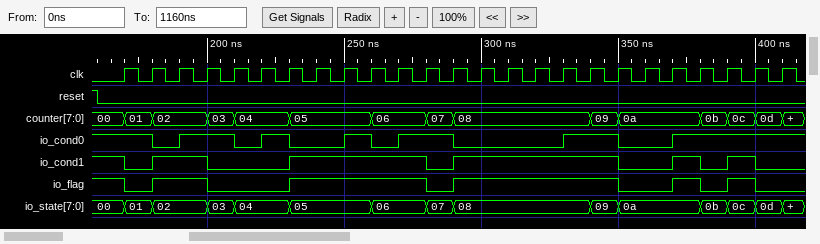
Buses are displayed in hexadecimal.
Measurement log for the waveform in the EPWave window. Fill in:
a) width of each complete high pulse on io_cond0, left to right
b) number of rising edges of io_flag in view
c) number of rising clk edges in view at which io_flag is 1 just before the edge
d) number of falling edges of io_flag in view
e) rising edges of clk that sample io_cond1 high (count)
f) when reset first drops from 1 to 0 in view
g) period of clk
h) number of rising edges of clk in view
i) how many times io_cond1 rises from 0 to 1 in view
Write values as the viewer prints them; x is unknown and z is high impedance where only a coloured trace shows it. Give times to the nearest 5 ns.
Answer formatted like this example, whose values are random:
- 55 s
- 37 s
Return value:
- 20 ns, 10 ns, 10 ns, 20 ns, 20 ns
- 5
- 16
- 6
- 16
- 160 ns
- 10 ns
- 25
- 5
